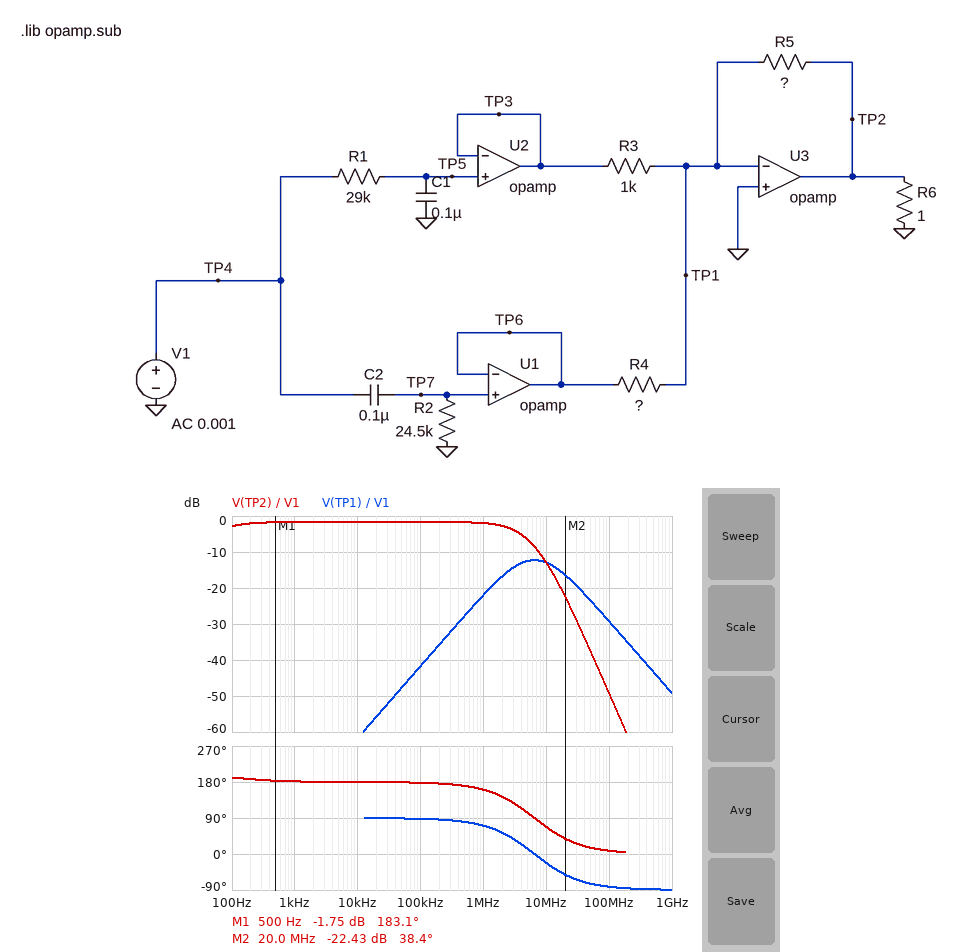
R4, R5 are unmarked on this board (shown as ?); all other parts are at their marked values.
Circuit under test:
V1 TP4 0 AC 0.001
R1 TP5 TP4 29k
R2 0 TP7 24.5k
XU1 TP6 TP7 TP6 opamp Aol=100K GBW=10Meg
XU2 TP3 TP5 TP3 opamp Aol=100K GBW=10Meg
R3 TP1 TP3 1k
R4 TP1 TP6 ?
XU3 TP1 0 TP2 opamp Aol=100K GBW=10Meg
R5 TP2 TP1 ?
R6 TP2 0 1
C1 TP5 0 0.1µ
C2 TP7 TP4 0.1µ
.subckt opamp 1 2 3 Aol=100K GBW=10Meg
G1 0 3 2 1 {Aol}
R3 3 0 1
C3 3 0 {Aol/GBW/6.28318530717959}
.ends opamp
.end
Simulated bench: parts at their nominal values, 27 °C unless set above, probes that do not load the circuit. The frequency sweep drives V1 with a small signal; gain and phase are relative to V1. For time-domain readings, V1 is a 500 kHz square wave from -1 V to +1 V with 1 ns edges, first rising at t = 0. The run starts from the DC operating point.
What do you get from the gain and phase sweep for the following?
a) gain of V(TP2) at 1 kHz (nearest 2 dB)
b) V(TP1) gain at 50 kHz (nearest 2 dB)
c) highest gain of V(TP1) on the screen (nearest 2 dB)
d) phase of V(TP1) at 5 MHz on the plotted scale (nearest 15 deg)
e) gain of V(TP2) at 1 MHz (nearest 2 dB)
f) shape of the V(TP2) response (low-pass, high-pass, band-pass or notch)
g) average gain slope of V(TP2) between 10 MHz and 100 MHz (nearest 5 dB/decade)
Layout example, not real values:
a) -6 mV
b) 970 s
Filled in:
a) -2 dB
b) -48 dB
c) -12 dB
d) 15 deg
e) -2 dB
f) low-pass
g) -35 dB/decade
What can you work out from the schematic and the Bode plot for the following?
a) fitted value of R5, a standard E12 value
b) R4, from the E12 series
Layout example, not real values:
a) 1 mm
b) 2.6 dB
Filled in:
a) 560 Ω
b) 680 Ω
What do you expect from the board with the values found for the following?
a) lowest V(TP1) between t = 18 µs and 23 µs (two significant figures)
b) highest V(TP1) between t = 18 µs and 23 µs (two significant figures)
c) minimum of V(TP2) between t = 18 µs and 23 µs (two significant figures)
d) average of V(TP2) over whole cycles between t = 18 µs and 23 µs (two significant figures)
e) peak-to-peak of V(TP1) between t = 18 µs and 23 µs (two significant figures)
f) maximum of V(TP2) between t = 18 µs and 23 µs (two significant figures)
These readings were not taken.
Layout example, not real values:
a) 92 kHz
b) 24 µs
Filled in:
a) -370 mV
b) 370 mV
c) -1.1 V
d) -260 mV
e) 740 mV
f) 560 mV
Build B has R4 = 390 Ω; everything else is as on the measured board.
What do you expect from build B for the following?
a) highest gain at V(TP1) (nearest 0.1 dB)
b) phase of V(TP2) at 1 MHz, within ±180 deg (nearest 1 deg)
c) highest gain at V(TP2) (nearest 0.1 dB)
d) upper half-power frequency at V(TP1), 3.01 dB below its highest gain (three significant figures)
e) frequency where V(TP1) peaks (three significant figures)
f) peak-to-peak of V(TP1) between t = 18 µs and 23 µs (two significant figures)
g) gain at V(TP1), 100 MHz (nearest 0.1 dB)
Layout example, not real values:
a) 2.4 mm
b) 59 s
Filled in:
a) -8.9 dB
b) 158 deg
c) 3.1 dB
d) 15.5 MHz
e) 5.78 MHz
f) 1.1 V
g) -26.4 dB
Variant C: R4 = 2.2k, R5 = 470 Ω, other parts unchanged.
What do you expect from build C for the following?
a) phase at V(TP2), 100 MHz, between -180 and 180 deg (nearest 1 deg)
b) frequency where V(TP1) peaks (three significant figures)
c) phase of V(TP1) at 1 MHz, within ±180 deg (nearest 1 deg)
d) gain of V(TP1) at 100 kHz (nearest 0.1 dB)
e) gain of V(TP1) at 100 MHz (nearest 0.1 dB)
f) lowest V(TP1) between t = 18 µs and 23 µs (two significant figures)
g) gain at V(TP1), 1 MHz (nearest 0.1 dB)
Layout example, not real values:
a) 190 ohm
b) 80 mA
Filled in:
a) 9 deg
b) 7.71 MHz
c) 75 deg
d) -53.4 dB
e) -38.0 dB
f) -120 mV
g) -33.6 dB
